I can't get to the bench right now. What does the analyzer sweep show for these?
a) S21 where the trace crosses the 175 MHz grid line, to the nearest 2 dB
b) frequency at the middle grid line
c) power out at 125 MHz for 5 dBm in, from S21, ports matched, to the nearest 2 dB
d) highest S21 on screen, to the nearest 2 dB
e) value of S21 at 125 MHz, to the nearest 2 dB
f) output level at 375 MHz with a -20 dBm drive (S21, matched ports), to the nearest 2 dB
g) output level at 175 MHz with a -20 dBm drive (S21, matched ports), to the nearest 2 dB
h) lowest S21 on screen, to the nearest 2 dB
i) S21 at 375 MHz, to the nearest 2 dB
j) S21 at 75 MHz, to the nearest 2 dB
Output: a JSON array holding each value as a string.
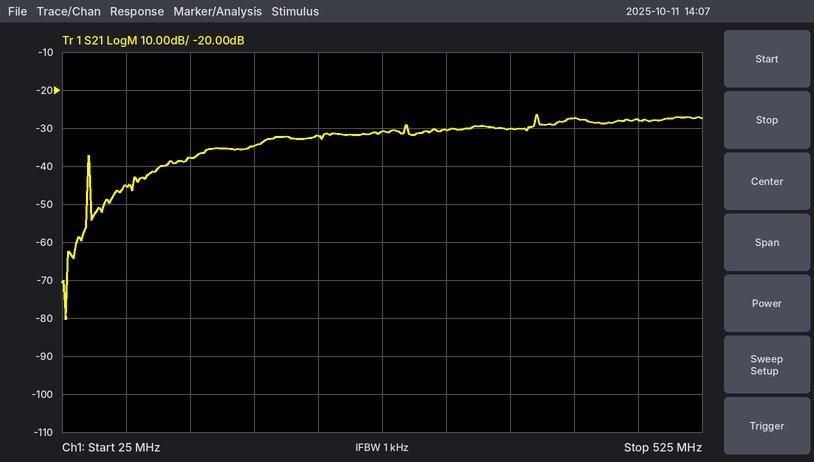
["-34 dB", "275 MHz", "-32 dBm", "-26 dB", "-38 dB", "-50 dBm", "-54 dBm", "-80 dB", "-30 dB", "-46 dB"]
